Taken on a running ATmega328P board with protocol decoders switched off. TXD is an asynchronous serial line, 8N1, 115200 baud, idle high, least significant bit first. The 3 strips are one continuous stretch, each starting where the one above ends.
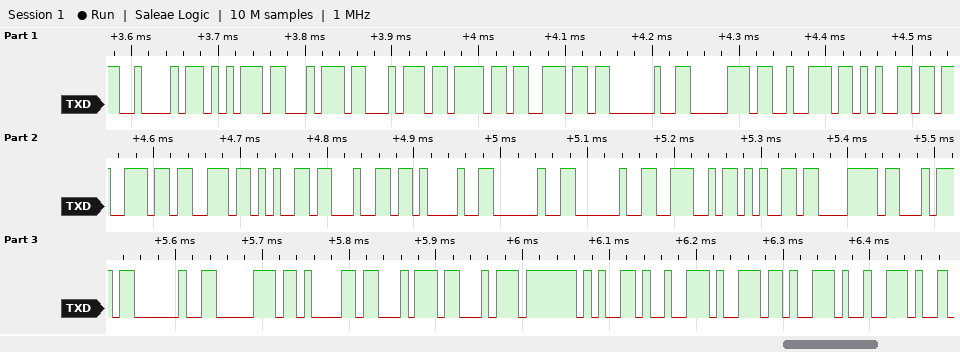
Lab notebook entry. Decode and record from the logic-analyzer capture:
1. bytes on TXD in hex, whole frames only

0x42 0x75 0x74 0x74 0x6F 0x6E 0x20 0x70 0x72 0x65 0x73 0x73 0x65 0x64 0x21 0x20 0x20 0x4E 0x65 0x78 0x74 0x20 0x70 0x61 0x74 0x74 0x65 0x72 0x6E 0x2E 0x2E
